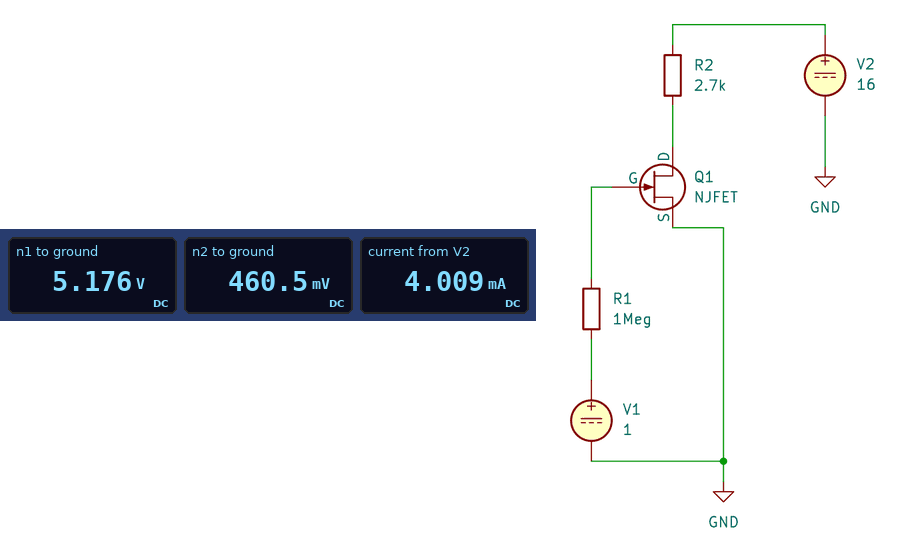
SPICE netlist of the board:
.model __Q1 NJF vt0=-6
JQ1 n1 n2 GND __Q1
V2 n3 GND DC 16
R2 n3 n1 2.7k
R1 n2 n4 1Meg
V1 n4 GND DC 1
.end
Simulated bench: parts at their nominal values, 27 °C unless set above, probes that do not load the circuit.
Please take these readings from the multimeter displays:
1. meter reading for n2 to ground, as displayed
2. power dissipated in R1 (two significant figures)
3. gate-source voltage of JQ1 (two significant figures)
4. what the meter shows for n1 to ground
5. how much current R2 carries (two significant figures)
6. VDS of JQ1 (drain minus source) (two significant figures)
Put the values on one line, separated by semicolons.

460.5 mV; 290 nW; 460 mV; 5.176 V; 4.0 mA; 5.2 V
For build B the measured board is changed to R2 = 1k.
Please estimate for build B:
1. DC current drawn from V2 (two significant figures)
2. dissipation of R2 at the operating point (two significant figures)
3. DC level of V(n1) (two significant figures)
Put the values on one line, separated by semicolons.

4.2 mA; 17 mW; 12 V
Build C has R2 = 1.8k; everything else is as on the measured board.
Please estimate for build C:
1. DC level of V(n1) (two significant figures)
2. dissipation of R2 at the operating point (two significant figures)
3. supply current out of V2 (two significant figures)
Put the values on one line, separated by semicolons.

8.5 V; 31 mW; 4.2 mA
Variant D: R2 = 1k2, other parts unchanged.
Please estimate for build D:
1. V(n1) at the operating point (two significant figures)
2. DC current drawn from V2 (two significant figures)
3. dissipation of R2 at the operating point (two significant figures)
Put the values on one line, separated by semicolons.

11 V; 4.2 mA; 21 mW
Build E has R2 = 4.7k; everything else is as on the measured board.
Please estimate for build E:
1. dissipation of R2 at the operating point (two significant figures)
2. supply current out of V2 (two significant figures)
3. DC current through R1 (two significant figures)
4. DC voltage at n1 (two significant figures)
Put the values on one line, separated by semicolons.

37 mW; 2.8 mA; 540 nA; 2.8 V
